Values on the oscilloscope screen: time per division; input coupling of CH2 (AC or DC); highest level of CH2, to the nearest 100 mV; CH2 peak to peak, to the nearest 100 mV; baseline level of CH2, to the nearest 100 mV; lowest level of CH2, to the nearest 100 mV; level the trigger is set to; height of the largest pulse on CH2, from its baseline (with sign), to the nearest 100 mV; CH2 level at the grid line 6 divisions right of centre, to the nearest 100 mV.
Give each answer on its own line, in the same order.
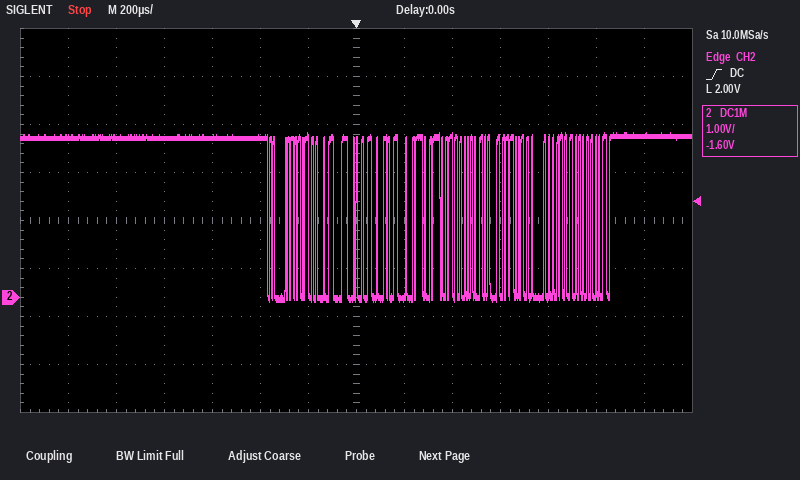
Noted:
200 µs
DC
3.4 V
3.5 V
3.3 V
-100 mV
2.00 V
-3.4 V
3.4 V
